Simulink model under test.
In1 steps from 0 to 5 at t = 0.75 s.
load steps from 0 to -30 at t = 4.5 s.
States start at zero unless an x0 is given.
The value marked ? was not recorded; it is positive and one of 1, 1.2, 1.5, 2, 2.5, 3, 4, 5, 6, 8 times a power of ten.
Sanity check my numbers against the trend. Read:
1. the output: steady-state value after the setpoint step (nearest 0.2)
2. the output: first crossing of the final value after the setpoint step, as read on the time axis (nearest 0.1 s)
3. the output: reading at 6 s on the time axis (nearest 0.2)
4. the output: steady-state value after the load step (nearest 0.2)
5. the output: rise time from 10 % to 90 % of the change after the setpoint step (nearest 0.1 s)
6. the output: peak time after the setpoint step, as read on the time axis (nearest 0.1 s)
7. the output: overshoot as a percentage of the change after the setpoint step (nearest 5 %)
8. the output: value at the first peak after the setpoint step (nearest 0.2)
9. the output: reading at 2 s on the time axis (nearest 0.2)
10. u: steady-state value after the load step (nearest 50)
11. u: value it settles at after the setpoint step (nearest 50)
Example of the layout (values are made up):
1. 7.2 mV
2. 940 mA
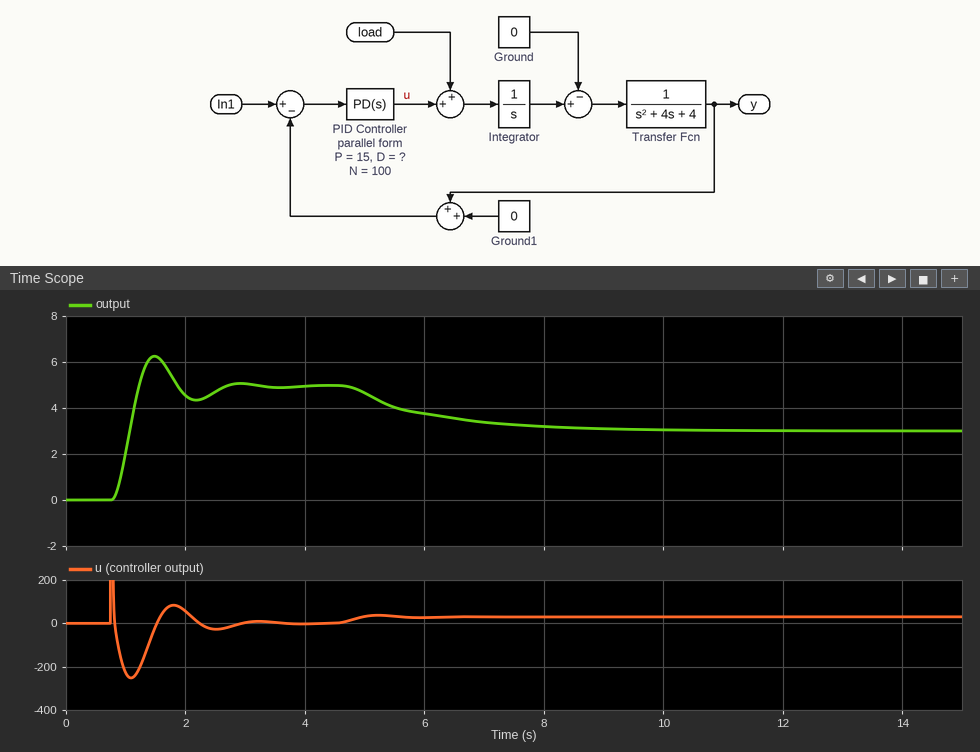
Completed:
1. 5.0
2. 1.2 s
3. 3.8
4. 3.0
5. 0.3 s
6. 1.5 s
7. 25 %
8. 6.2
9. 4.6
10. 50
11. 0
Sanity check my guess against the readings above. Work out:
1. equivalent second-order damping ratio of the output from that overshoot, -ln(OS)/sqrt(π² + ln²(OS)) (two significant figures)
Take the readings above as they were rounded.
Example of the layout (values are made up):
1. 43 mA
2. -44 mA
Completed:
1. 0.40
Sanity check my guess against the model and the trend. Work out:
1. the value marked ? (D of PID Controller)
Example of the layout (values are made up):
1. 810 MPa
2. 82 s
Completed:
1. 20
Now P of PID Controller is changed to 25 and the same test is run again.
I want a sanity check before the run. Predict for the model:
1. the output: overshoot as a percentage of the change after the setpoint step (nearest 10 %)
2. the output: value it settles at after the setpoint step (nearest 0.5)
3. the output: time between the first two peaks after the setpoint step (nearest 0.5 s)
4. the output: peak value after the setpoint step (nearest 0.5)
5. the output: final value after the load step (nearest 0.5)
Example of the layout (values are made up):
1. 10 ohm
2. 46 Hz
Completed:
1. 40 %
2. 5.0
3. 1.5 s
4. 7.0
5. 4.0
